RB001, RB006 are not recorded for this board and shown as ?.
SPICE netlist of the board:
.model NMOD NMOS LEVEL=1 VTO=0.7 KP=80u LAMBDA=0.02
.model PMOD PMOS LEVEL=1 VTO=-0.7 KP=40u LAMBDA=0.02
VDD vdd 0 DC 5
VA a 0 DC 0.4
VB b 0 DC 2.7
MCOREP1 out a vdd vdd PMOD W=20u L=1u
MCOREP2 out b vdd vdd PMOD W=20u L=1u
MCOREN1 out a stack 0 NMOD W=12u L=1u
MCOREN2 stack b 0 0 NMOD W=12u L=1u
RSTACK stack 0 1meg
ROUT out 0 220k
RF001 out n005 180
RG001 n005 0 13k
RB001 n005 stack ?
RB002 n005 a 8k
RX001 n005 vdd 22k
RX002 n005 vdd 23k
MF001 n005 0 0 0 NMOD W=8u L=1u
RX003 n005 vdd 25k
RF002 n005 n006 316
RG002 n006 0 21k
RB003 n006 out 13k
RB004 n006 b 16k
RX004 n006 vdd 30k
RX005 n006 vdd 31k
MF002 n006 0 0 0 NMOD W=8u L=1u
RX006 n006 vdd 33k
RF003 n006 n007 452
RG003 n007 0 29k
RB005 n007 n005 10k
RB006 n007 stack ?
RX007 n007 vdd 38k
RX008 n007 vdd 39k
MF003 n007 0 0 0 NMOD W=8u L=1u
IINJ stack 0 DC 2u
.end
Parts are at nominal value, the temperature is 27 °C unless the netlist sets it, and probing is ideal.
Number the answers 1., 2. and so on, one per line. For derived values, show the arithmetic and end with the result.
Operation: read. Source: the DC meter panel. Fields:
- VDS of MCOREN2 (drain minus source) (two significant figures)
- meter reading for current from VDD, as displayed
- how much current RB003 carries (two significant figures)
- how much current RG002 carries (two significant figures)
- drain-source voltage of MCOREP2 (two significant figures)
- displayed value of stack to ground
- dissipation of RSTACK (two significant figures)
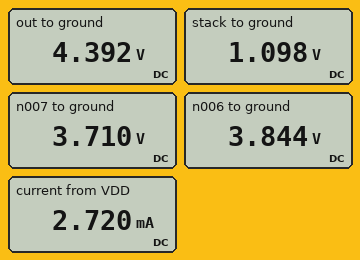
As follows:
1. 1.098 V = 1.1 V
2. 2.720 mA
3. (4.392 V - 3.844 V) / 13 kΩ = 42 µA
4. (3.844 V) / 21 kΩ = 180 µA
5. 4.392 V - 5 V = -610 mV
6. 1.098 V
7. (1.098 V)^2 / 1 MΩ = 1.2 µW
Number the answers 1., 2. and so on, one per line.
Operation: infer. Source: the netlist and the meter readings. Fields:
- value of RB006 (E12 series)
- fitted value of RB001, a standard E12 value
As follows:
1. 10 kΩ
2. 2.2 kΩ
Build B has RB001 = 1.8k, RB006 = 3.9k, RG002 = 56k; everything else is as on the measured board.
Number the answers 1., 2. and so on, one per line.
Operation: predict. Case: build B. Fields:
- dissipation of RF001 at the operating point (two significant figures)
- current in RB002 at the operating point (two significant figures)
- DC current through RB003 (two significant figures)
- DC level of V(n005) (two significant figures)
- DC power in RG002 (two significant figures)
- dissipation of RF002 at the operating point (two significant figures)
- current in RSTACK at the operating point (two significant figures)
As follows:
1. 1.1 mW
2. 440 µA
3. 46 µA
4. 3.9 V
5. 250 µW
6. 76 µW
7. 1.5 µA
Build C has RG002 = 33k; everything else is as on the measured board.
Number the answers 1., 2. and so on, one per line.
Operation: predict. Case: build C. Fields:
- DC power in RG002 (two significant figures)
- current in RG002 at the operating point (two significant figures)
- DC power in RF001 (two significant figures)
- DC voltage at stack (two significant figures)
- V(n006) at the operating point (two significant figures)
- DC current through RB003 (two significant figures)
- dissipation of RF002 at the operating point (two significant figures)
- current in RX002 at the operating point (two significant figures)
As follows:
1. 460 µW
2. 120 µA
3. 960 µW
4. 1.1 V
5. 3.9 V
6. 40 µA
7. 38 µW
8. 44 µA
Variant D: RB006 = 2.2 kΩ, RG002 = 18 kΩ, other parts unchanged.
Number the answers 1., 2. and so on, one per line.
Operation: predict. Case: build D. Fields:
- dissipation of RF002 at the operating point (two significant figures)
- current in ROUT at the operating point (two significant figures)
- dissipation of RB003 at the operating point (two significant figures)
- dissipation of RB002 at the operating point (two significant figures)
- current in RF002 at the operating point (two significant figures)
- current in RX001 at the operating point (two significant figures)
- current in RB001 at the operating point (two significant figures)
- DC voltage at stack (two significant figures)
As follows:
1. 220 µW
2. 20 µA
3. 40 µW
4. 1.5 mW
5. 830 µA
6. 51 µA
7. 1.1 mA
8. 1.5 V
